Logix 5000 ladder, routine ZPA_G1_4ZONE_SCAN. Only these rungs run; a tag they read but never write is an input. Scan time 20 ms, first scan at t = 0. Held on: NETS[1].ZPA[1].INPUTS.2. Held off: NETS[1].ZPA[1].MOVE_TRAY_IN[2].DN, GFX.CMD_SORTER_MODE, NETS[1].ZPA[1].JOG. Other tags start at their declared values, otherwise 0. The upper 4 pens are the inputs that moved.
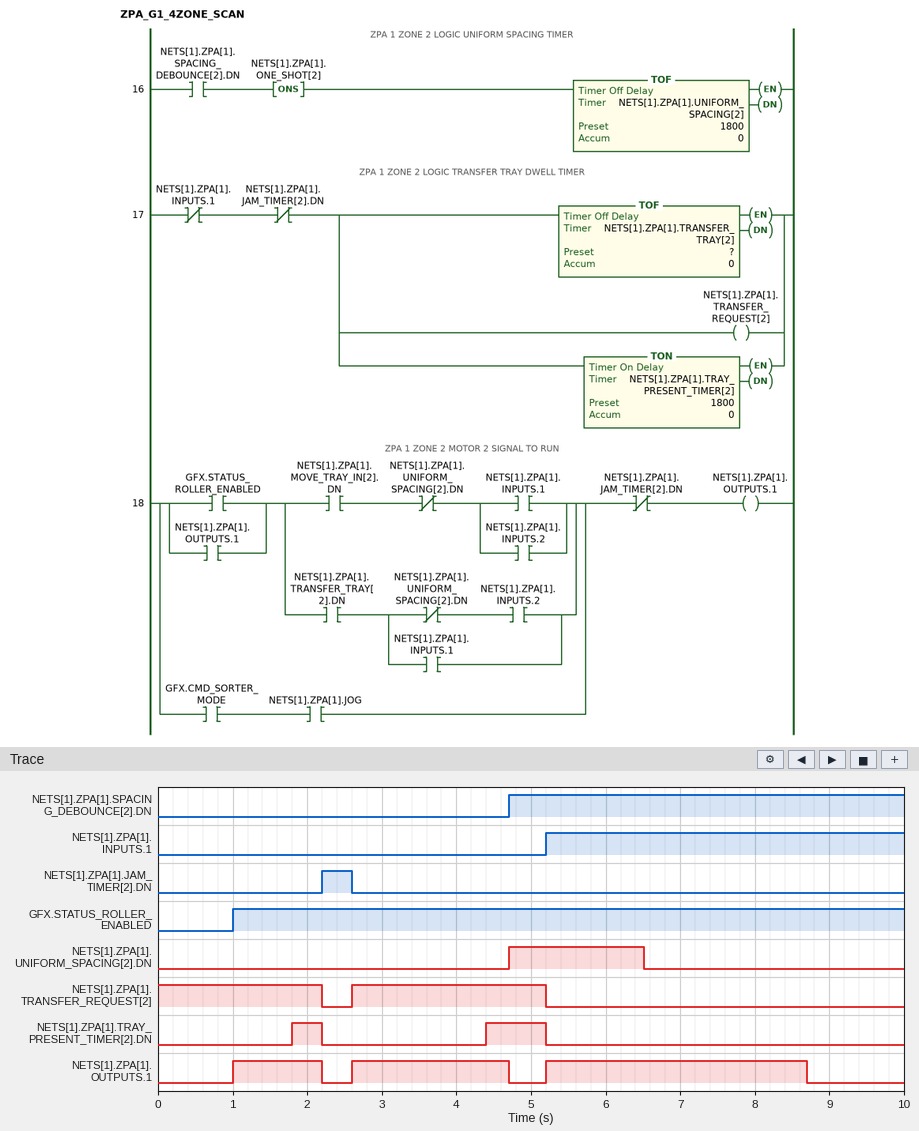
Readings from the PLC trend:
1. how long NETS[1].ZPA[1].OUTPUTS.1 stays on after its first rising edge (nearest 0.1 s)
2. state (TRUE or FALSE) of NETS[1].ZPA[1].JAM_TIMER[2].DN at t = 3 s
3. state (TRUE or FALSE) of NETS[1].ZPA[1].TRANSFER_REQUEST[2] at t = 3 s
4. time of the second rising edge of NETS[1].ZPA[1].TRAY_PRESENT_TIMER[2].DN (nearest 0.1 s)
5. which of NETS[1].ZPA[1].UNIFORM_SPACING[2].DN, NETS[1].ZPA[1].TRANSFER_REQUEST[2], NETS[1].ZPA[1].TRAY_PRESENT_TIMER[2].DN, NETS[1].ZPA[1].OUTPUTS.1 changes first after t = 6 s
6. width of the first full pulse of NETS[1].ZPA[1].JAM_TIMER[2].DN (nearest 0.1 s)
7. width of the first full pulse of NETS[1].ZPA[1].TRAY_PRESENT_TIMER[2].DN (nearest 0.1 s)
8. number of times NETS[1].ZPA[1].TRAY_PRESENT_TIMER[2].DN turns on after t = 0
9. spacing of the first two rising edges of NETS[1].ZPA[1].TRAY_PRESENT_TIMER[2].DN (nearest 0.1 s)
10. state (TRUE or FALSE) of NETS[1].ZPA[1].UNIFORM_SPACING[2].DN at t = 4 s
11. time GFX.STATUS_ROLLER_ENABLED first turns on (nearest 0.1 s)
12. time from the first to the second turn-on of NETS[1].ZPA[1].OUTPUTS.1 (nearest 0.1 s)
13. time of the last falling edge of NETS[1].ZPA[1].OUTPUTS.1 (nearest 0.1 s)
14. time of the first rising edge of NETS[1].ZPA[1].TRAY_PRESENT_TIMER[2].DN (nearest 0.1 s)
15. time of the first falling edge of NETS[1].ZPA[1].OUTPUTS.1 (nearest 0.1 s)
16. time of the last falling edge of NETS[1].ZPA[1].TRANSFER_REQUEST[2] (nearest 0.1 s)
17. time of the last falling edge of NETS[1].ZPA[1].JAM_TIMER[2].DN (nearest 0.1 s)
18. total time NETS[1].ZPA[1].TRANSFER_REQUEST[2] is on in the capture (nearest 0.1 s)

1.2 s
FALSE
TRUE
4.4 s
NETS[1].ZPA[1].UNIFORM_SPACING[2].DN
0.4 s
0.4 s
2
2.6 s
FALSE
1.0 s
1.6 s
8.7 s
1.8 s
2.2 s
5.2 s
2.6 s
4.8 s
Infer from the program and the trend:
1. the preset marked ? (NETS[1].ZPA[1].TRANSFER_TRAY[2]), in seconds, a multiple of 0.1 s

3.5 s
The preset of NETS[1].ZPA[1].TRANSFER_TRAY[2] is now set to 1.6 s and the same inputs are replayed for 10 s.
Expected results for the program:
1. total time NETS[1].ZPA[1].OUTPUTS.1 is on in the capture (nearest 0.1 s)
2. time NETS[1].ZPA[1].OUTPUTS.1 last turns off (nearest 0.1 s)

4.9 s
6.8 s
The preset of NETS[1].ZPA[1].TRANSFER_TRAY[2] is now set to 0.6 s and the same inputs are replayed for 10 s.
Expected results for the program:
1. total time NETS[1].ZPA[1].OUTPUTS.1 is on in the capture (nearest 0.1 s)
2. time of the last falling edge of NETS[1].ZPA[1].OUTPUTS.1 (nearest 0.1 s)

3.9 s
5.8 s
